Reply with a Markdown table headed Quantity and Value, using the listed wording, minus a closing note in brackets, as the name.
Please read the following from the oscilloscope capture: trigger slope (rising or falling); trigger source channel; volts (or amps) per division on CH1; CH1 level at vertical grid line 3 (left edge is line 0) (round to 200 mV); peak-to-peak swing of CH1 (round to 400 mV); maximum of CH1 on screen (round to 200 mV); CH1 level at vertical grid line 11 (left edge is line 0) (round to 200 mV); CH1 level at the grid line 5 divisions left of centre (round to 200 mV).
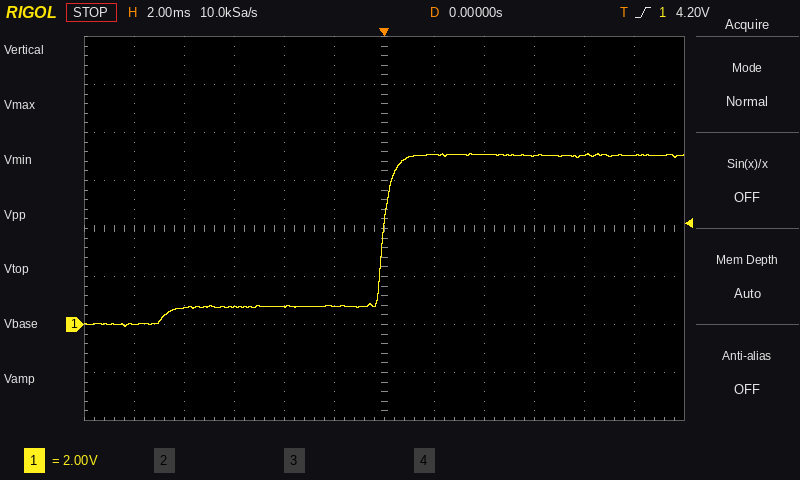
| Quantity | Value |
|---|---|
| trigger slope | rising |
| trigger source channel | CH1 |
| volts (or amps) per division on CH1 | 2 V |
| CH1 level at vertical grid line 3 (left edge is line 0) | 800 mV |
| peak-to-peak swing of CH1 | 7.2 V |
| maximum of CH1 on screen | 7.2 V |
| CH1 level at vertical grid line 11 (left edge is line 0) | 7.0 V |
| CH1 level at the grid line 5 divisions left of centre | 0.0 V |
